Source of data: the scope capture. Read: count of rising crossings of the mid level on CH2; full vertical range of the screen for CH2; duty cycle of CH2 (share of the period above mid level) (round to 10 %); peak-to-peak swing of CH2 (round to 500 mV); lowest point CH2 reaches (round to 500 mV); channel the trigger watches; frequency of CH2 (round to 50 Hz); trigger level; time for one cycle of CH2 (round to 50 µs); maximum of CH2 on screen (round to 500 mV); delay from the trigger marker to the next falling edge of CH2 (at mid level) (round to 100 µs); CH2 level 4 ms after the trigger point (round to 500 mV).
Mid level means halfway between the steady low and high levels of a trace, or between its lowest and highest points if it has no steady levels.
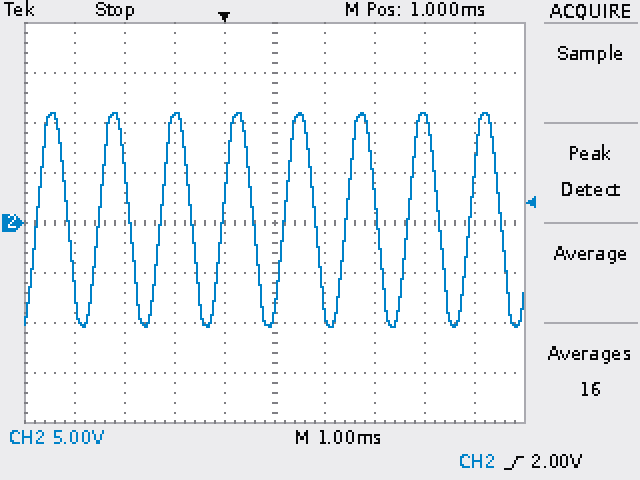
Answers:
8
40 V
50 %
21.5 V
-10.5 V
CH2
800 Hz
2.00 V
1.25 ms
11.0 V
600 µs
10.5 V
